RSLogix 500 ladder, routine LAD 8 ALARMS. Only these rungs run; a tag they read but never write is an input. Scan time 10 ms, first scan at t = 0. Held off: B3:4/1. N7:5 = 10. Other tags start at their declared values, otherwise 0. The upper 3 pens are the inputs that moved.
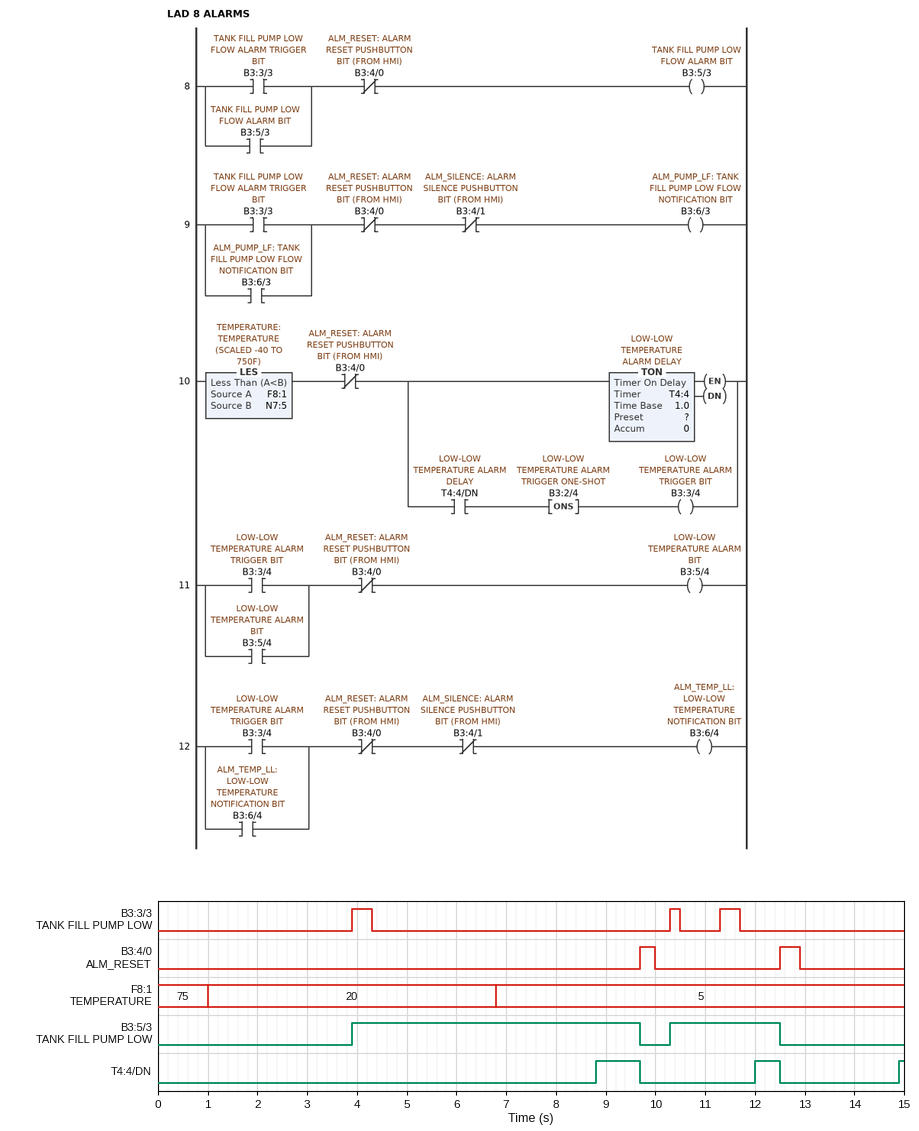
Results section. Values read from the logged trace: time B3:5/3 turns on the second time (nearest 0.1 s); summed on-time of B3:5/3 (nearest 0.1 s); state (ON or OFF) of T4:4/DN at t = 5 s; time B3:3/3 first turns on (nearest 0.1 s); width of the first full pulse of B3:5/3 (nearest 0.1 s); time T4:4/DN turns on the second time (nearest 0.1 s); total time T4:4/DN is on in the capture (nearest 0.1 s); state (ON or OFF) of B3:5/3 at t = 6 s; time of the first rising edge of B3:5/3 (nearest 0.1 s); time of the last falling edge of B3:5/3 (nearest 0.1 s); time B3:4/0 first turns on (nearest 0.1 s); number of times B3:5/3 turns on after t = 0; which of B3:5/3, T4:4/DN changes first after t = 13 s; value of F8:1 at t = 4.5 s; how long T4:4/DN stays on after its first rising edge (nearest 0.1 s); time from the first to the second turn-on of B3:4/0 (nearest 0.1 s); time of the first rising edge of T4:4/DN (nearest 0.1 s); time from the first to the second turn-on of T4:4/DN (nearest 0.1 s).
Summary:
10.3 s
8.0 s
OFF
3.9 s
5.8 s
12.0 s
1.5 s
ON
3.9 s
12.5 s
9.7 s
2
T4:4/DN
20
0.9 s
2.8 s
8.8 s
3.2 s
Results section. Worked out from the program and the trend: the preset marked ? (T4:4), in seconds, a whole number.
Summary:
2 s
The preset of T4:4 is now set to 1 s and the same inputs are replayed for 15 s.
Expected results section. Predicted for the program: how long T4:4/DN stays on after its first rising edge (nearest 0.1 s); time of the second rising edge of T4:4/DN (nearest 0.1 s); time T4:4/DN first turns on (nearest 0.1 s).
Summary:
1.9 s
11.0 s
7.8 s
